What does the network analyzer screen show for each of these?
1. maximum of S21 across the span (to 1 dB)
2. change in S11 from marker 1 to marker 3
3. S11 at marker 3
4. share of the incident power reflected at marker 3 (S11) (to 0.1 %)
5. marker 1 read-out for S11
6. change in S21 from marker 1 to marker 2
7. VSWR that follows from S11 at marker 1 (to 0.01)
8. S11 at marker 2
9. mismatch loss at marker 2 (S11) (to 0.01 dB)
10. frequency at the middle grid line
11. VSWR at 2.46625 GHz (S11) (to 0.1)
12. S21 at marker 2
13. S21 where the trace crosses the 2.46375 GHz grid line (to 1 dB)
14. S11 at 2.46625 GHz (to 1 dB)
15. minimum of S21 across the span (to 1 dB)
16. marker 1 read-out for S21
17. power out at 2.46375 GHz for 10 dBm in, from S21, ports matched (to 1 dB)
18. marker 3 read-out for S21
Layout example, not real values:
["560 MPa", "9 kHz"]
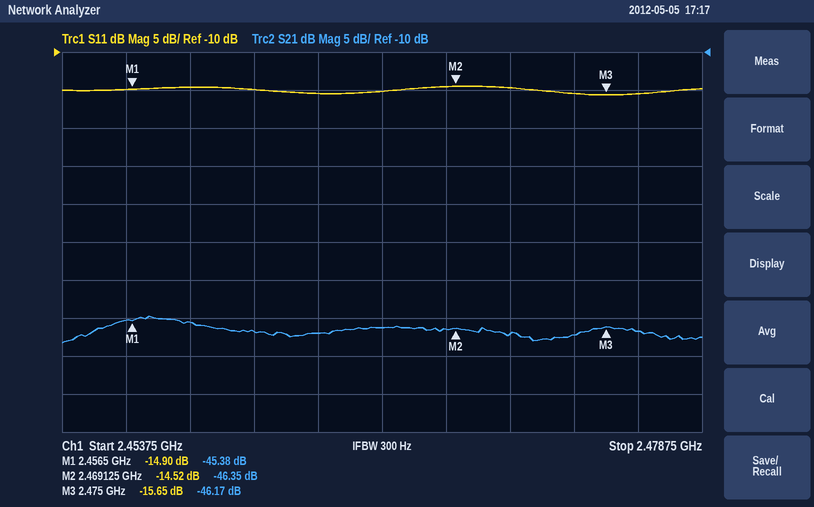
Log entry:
["-45 dB", "-0.75 dB", "-15.65 dB", "2.7 %", "-14.90 dB", "-0.97 dB", "1.44", "-14.52 dB", "0.16 dB", "2.46625 GHz", "1.4", "-46.35 dB", "-47 dB", "-15 dB", "-48 dB", "-45.38 dB", "-37 dBm", "-46.17 dB"]
